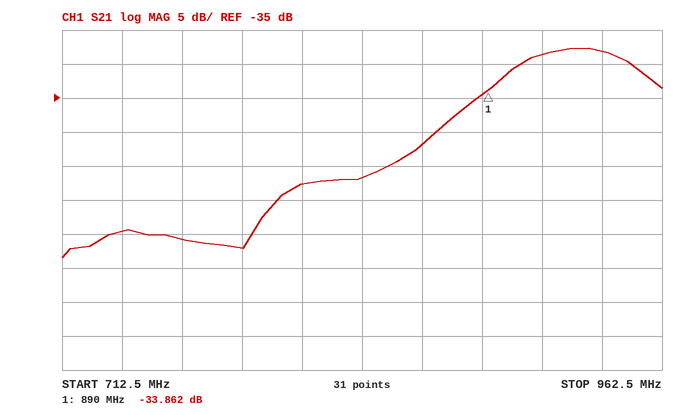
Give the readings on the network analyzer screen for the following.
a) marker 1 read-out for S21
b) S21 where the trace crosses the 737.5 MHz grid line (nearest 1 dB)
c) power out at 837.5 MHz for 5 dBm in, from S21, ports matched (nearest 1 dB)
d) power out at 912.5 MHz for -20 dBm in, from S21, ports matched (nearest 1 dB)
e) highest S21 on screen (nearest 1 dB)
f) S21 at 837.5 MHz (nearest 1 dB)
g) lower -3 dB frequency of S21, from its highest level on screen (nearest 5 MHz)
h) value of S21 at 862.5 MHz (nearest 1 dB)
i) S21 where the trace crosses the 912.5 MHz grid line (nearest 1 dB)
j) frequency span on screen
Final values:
-33.862 dB
-55 dB
-42 dBm
-49 dBm
-28 dB
-47 dB
900 MHz
-42 dB
-29 dB
250 MHz
